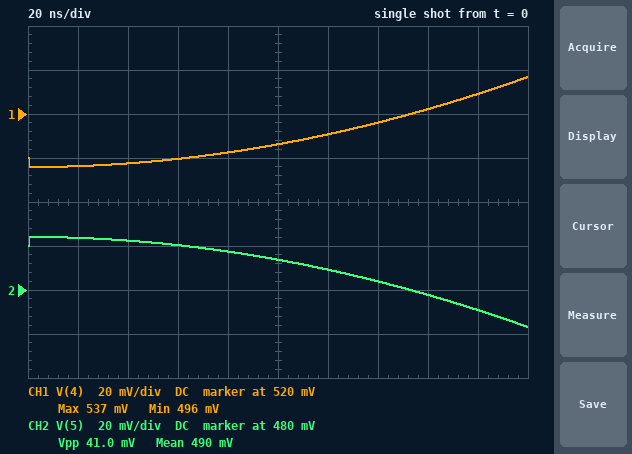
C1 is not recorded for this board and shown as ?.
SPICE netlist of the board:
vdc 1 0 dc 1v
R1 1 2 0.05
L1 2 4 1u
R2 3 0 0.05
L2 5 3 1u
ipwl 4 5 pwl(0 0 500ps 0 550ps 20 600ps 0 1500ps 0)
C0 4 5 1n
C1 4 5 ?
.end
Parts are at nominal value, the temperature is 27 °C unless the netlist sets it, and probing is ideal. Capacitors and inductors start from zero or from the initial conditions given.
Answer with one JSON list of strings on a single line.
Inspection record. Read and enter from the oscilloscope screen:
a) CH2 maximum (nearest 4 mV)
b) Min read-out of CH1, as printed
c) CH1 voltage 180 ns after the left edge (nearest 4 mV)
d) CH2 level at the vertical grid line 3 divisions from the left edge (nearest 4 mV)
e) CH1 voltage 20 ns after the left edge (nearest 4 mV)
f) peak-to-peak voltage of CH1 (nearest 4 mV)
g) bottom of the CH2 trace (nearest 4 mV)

["504 mV", "496 mV", "528 mV", "500 mV", "496 mV", "40 mV", "464 mV"]
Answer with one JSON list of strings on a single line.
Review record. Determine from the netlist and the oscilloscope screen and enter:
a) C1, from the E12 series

["120 nF"]
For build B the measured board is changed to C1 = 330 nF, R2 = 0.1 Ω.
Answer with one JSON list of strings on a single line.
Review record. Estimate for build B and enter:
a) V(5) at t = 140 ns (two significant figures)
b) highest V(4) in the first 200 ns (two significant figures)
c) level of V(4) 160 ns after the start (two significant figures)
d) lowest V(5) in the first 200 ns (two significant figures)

["500 mV", "520 mV", "510 mV", "490 mV"]
